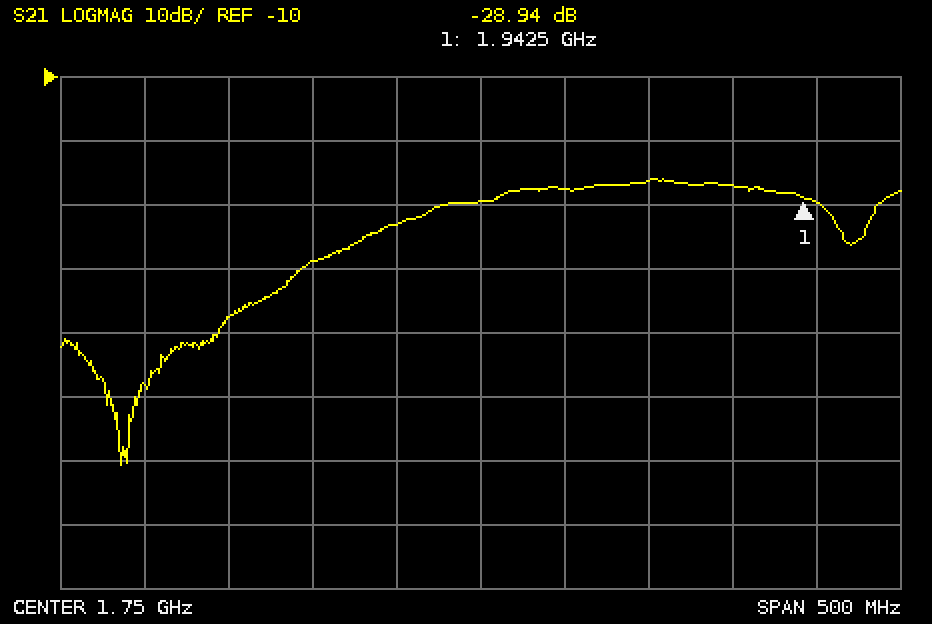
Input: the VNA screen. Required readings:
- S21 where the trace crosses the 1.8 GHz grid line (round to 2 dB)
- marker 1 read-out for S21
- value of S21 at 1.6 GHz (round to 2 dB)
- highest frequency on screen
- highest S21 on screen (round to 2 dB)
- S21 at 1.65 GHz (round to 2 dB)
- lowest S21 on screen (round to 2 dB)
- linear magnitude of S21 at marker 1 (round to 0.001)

-28 dB
-28.94 dB
-48 dB
2 GHz
-26 dB
-38 dB
-70 dB
0.036
